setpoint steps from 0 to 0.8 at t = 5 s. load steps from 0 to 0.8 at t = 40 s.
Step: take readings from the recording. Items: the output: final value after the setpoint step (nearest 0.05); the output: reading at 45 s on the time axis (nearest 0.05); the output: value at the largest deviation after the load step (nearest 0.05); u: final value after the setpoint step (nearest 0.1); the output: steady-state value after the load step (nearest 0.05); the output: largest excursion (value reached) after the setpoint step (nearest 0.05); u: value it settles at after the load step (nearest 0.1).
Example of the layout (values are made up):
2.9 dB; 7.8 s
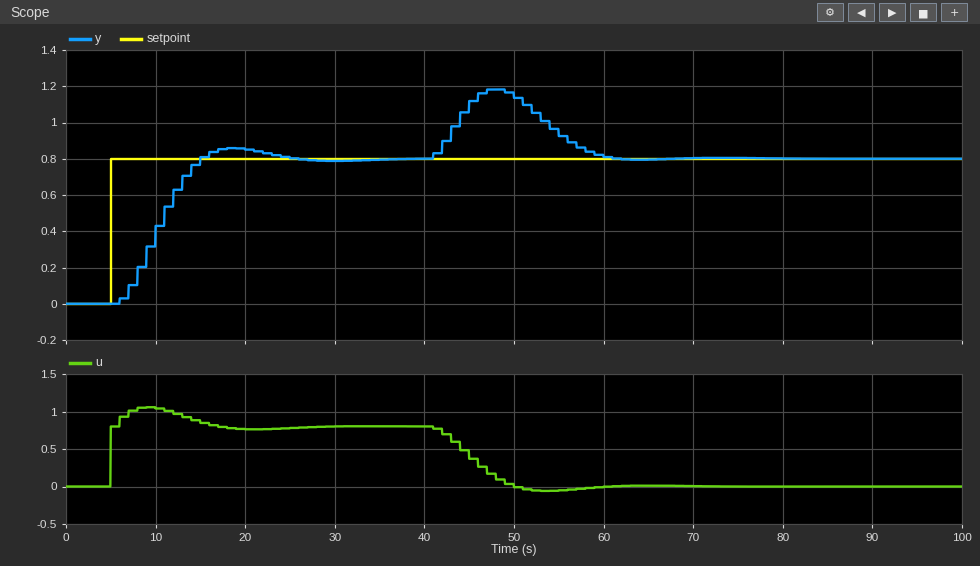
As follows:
0.80; 1.10; 1.20; 0.8; 0.80; 0.85; 0.0
